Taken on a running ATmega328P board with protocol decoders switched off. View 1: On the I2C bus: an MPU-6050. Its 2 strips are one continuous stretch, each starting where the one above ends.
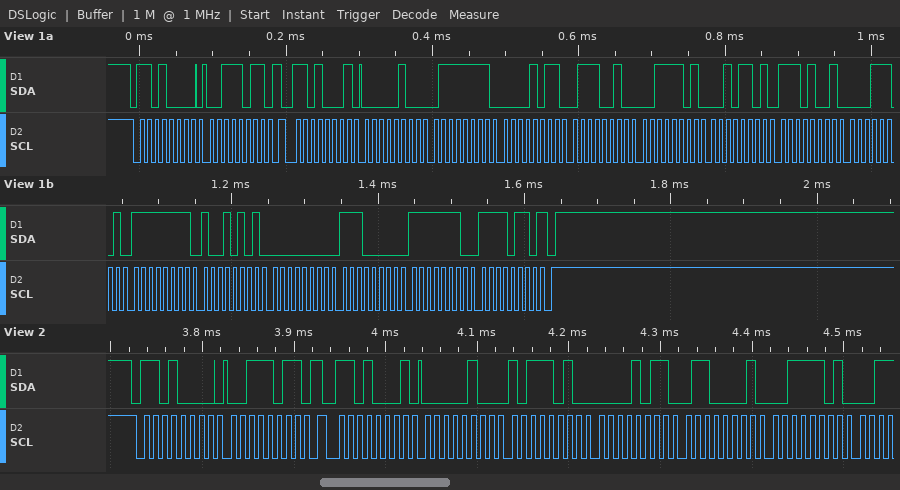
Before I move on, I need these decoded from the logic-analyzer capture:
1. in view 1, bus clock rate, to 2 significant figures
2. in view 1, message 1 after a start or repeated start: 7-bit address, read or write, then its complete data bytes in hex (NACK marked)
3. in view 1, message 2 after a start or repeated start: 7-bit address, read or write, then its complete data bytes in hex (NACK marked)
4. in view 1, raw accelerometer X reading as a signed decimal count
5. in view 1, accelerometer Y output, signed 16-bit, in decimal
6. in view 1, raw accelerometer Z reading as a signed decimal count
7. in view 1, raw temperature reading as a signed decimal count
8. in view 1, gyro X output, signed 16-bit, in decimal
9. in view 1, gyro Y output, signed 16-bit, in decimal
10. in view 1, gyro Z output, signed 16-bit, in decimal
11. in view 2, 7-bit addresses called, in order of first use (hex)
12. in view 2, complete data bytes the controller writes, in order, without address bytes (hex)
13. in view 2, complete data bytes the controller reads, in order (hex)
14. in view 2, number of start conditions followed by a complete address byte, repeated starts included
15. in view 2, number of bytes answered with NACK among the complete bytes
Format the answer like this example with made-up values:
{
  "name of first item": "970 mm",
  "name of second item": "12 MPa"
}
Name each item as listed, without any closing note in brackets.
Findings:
{
  "in view 1, bus clock rate, to 2 significant figures": "100 kHz",
  "in view 1, message 1 after a start or repeated start: 7-bit address, read or write, then its complete data bytes in hex": "0x68 write: 3B",
  "in view 1, message 2 after a start or repeated start: 7-bit address, read or write, then its complete data bytes in hex": "0x68 read: 04 7F 0B 72 3D 2D E9 1D FF 95 00 E0 FE F6 NACK",
  "in view 1, raw accelerometer X reading as a signed decimal count": "1151",
  "in view 1, accelerometer Y output, signed 16-bit, in decimal": "2930",
  "in view 1, raw accelerometer Z reading as a signed decimal count": "15661",
  "in view 1, raw temperature reading as a signed decimal count": "-5859",
  "in view 1, gyro X output, signed 16-bit, in decimal": "-107",
  "in view 1, gyro Y output, signed 16-bit, in decimal": "224",
  "in view 1, gyro Z output, signed 16-bit, in decimal": "-266",
  "in view 2, 7-bit addresses called, in order of first use": "0x68",
  "in view 2, complete data bytes the controller writes, in order, without address bytes": "3B",
  "in view 2, complete data bytes the controller reads, in order": "04 BA 0B 61 3D",
  "in view 2, number of start conditions followed by a complete address byte, repeated starts included": "2",
  "in view 2, number of bytes answered with NACK among the complete bytes": "0"
}
